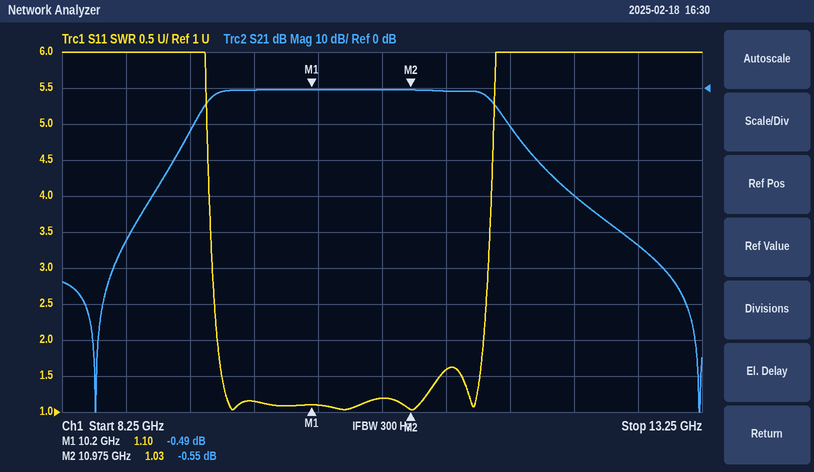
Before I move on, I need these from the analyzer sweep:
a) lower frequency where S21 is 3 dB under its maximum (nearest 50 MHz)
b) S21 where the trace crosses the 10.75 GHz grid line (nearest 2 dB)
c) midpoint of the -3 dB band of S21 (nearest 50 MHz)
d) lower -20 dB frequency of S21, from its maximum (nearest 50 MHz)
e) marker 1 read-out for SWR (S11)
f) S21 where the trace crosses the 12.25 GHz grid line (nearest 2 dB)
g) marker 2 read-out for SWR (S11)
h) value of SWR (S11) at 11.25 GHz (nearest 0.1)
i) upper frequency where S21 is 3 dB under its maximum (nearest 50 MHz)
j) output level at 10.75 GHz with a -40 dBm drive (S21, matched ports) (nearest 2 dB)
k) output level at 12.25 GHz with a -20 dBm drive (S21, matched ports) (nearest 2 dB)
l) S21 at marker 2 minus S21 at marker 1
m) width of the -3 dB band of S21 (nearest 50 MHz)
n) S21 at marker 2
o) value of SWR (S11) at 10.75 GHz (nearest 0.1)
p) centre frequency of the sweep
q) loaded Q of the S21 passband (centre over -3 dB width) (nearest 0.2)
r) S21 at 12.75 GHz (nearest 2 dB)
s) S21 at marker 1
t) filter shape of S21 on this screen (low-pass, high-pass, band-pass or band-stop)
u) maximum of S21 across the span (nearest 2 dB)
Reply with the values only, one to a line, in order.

9.40 GHz
0 dB
10.50 GHz
9.10 GHz
1.10
-30 dB
1.03
1.6
11.60 GHz
-40 dBm
-50 dBm
-0.06 dB
2.20 GHz
-0.55 dB
1.2
10.75 GHz
4.8
-44 dB
-0.49 dB
band-pass
0 dB
